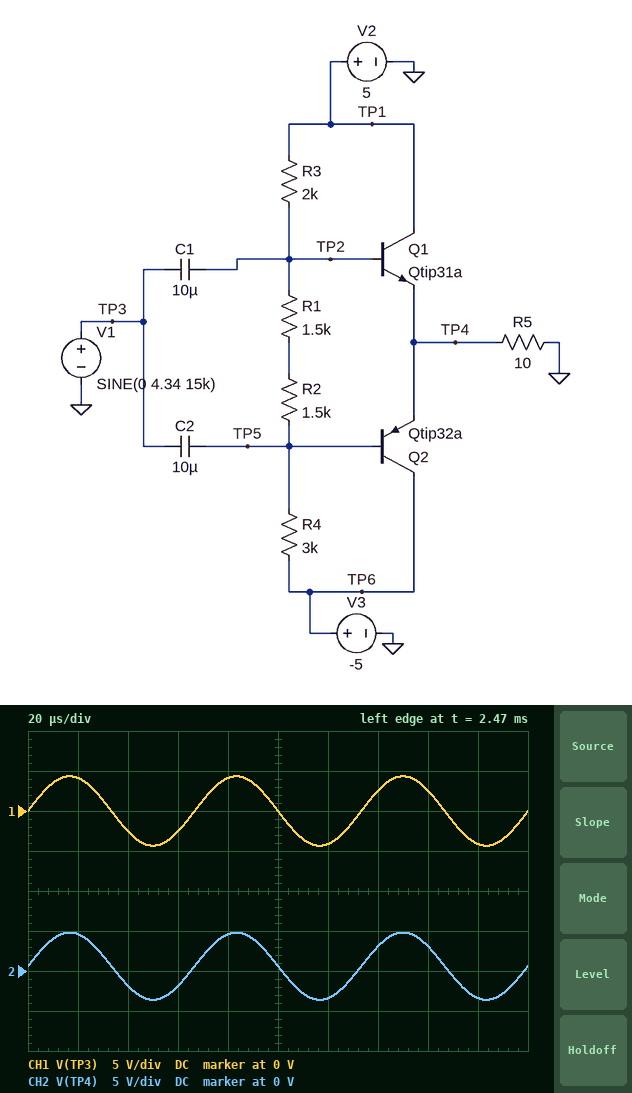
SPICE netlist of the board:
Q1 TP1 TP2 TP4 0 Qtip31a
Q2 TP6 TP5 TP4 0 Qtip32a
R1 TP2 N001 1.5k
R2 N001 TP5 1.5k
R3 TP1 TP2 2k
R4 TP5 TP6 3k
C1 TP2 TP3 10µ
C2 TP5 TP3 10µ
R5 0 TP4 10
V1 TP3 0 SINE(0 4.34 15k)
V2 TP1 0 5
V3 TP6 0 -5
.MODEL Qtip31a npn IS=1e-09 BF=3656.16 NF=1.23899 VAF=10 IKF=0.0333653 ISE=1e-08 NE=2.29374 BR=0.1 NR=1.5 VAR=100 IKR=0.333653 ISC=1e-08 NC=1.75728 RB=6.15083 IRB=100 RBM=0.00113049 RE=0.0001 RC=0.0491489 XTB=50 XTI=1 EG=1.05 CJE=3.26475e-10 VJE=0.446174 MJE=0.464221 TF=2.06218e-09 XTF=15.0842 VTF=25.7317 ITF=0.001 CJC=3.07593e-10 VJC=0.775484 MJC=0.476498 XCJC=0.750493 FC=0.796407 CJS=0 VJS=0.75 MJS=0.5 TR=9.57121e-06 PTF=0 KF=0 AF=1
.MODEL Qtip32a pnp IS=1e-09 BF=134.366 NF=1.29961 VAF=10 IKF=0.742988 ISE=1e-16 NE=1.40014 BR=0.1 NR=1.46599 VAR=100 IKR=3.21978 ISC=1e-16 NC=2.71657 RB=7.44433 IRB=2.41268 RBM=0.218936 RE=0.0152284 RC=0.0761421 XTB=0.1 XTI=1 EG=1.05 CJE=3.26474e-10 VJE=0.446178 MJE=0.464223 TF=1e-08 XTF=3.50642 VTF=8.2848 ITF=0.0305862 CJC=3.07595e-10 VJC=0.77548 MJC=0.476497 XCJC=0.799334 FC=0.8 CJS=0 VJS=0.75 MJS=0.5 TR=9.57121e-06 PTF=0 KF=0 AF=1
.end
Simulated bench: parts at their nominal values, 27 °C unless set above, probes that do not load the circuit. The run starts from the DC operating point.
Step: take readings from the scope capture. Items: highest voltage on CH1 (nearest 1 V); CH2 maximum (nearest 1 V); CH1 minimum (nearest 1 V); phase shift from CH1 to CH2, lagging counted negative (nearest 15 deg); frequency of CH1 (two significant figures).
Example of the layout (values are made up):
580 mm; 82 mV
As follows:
4 V; 5 V; -4 V; 0 deg; 15 kHz
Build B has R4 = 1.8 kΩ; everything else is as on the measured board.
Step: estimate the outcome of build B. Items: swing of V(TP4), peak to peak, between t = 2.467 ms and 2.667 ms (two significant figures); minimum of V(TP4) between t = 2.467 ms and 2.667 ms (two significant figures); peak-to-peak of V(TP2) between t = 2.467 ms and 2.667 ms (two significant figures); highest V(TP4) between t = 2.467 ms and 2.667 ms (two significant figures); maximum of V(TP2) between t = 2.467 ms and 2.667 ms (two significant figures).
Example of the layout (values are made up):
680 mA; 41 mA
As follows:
8.5 V; -4.0 V; 8.7 V; 4.5 V; 5.2 V
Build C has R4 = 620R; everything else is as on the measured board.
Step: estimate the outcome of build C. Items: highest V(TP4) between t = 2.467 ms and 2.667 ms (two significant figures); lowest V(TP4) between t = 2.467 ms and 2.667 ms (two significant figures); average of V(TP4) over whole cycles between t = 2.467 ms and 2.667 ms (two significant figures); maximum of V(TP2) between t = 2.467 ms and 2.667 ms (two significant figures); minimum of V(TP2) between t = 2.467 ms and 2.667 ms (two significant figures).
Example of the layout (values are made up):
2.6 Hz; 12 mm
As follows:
3.5 V; -4.8 V; -730 mV; 4.3 V; -4.4 V
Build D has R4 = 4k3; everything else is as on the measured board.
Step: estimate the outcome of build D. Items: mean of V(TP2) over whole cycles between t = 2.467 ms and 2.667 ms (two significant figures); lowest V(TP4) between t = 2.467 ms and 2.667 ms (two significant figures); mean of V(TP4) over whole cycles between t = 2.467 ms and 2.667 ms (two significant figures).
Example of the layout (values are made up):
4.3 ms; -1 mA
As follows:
1.3 V; -3.3 V; 770 mV
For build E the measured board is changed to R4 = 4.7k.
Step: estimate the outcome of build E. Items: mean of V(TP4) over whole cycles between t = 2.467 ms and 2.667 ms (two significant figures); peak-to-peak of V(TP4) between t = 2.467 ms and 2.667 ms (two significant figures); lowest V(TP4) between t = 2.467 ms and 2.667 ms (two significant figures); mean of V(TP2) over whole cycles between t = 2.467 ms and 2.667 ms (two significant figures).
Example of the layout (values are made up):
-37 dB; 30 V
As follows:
810 mV; 8.0 V; -3.2 V; 1.3 V
